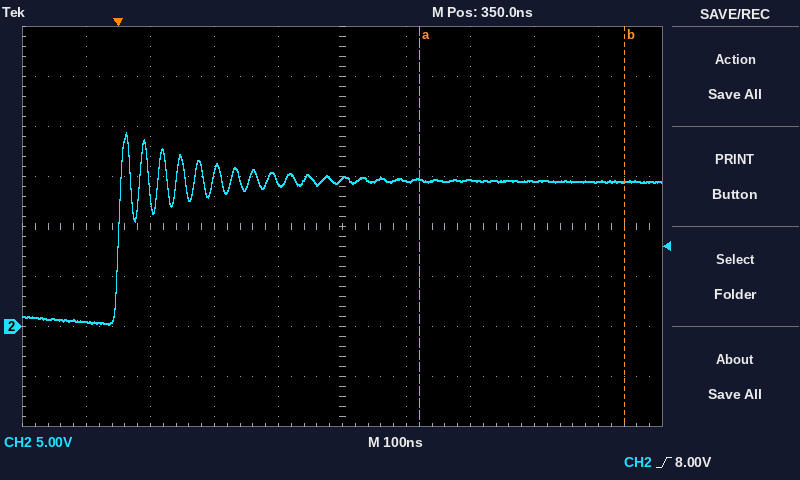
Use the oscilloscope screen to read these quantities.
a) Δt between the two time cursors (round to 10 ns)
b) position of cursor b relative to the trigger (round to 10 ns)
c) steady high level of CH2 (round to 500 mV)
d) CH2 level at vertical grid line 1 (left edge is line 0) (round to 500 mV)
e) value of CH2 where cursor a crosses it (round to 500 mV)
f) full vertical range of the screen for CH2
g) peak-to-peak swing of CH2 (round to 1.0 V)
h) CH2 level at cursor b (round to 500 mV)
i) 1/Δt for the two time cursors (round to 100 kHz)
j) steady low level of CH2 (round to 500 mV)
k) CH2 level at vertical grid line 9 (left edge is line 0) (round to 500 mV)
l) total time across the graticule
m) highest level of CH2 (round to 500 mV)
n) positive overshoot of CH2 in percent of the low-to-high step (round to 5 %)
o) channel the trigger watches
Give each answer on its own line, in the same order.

320 ns
+790 ns
14.5 V
500 mV
14.5 V
40 V
19.0 V
14.5 V
3.1 MHz
500 mV
14.5 V
1 µs
19.5 V
35 %
CH2
